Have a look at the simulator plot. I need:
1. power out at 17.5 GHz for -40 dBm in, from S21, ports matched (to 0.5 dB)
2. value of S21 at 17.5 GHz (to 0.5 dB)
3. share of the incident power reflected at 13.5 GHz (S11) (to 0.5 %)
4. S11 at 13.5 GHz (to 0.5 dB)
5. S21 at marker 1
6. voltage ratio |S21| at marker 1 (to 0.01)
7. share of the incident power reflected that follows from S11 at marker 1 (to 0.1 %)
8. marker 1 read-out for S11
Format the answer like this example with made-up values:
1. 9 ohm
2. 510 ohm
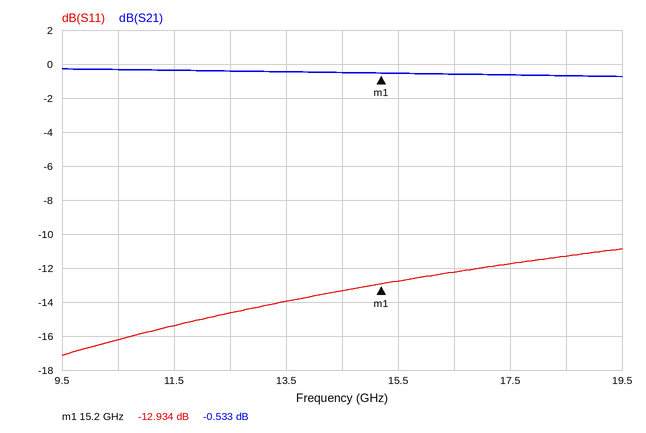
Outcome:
1. -40.5 dBm
2. -0.5 dB
3. 4.0 %
4. -14.0 dB
5. -0.533 dB
6. 0.94
7. 5.1 %
8. -12.934 dB
